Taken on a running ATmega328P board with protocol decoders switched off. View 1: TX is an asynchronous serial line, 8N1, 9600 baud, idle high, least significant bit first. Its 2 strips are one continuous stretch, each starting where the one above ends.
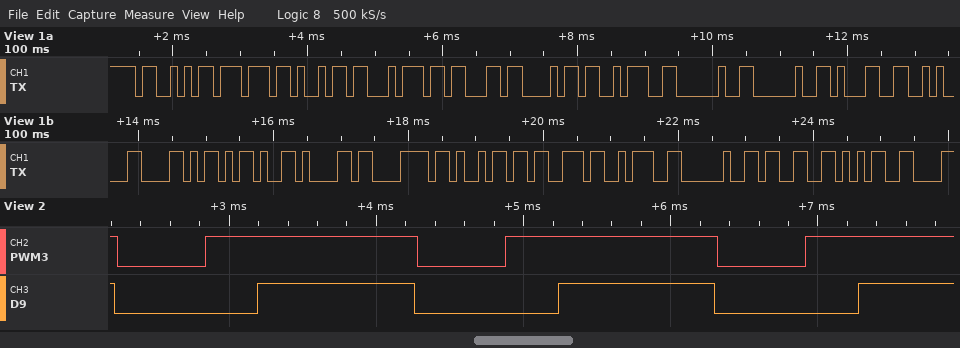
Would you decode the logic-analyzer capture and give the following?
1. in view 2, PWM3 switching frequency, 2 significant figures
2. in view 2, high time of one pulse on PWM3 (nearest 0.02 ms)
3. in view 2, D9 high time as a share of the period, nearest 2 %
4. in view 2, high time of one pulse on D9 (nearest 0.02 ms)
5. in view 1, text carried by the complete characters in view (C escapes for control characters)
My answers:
490 Hz
1.44 ms
52 %
1.06 ms
"Switch:  1\nX-axis: 35"
